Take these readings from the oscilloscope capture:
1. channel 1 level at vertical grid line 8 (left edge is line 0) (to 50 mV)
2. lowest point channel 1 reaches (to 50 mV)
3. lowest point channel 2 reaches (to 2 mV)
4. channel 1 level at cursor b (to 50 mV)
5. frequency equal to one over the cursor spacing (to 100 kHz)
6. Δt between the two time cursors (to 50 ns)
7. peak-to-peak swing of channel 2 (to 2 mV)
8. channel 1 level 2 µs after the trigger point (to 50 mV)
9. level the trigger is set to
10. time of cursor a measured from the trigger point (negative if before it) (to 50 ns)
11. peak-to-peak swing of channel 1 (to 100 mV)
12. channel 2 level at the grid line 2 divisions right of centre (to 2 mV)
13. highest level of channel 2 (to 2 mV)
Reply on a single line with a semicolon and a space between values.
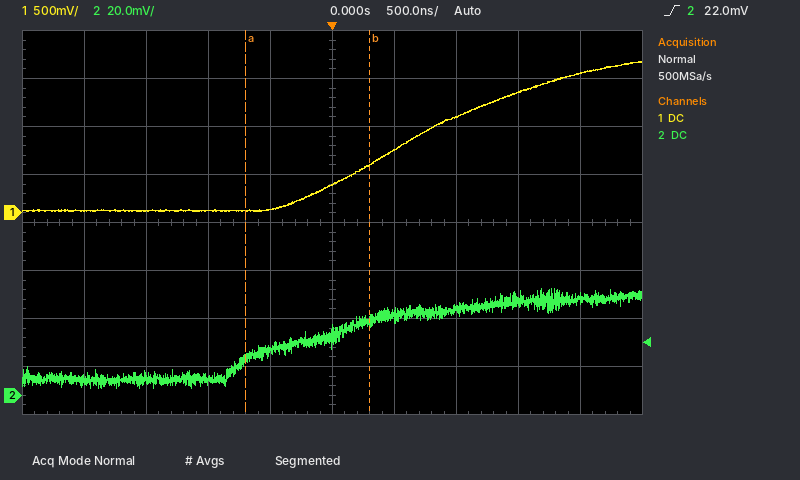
1.25 V; 0 mV; 2 mV; 500 mV; 1.0 MHz; 1.00 µs; 42 mV; 1.45 V; 22.0 mV; -700 ns; 1.60 V; 36 mV; 44 mV
